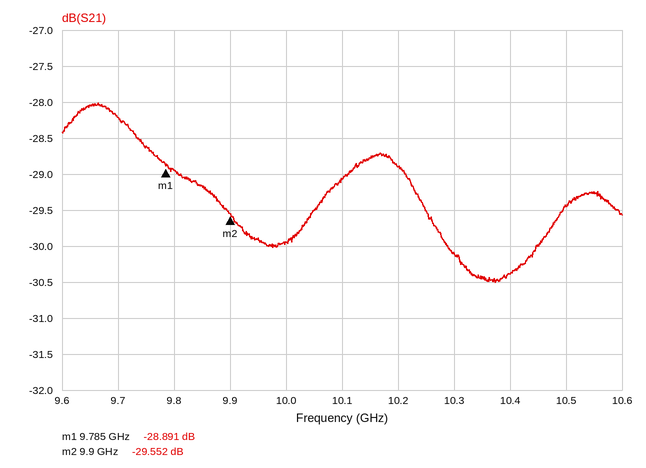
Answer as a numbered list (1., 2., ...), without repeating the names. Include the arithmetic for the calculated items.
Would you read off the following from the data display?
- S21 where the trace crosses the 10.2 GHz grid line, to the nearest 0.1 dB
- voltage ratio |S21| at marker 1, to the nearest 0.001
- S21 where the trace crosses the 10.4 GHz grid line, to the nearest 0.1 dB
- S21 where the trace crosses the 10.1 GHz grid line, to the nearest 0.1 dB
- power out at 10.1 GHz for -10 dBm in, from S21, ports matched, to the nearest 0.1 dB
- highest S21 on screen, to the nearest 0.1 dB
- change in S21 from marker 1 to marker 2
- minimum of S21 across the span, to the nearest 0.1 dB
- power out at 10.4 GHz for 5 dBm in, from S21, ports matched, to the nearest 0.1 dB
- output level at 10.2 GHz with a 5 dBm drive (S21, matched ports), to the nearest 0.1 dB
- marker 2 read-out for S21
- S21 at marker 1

1. -28.9 dB
2. 10^(-28.891/20) ≈ 0.036
3. -30.4 dB
4. -29.1 dB
5. -10 dBm + (-29.1 dB) = -39.1 dBm
6. -28.0 dB
7. -29.552 − (-28.891) = -0.661 dB
8. -30.5 dB
9. 5 dBm + (-30.4 dB) = -25.4 dBm
10. 5 dBm + (-28.9 dB) = -23.9 dBm
11. -29.552 dB
12. -28.891 dB
